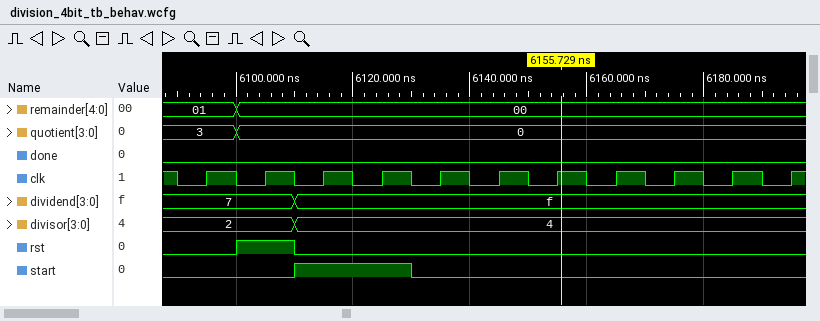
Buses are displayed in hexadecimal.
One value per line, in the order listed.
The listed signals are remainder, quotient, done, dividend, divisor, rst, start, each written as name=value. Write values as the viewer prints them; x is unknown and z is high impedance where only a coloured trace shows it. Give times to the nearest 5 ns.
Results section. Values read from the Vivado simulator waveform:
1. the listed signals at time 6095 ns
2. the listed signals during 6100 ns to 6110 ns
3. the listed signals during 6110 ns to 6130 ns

remainder=01, quotient=3, done=0, dividend=7, divisor=2, rst=0, start=0
remainder=00, quotient=0, done=0, dividend=7, divisor=2, rst=1, start=0
remainder=00, quotient=0, done=0, dividend=f, divisor=4, rst=0, start=1
